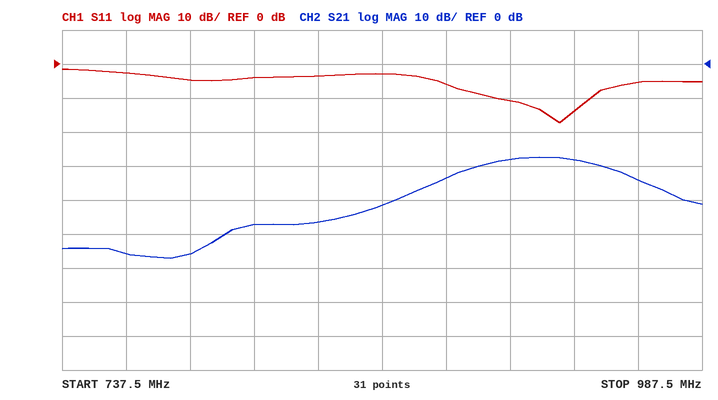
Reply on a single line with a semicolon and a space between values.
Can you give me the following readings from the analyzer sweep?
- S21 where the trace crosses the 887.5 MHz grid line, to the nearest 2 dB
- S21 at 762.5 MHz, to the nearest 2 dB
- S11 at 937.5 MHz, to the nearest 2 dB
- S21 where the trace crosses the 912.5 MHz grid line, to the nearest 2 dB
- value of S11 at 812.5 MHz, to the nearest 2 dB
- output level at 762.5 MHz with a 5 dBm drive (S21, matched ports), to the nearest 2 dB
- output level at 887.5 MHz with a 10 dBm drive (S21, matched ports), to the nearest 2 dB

-34 dB; -56 dB; -14 dB; -28 dB; -4 dB; -50 dBm; -24 dBm
